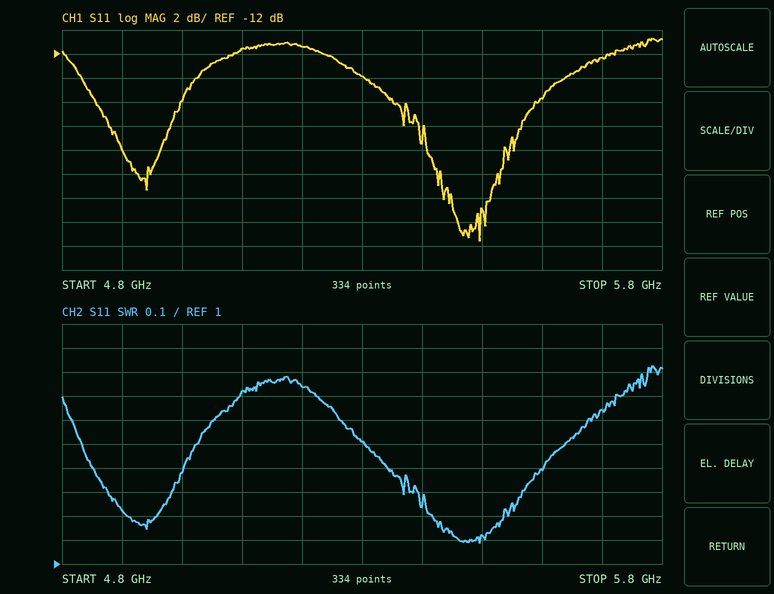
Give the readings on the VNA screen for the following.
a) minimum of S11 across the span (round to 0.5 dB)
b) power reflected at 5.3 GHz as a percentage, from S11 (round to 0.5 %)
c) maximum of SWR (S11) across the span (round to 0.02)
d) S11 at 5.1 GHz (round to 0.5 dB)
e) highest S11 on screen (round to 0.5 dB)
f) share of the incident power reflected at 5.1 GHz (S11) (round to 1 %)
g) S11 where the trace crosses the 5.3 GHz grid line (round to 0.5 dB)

-27.5 dB
4.0 %
1.82
-11.5 dB
-10.5 dB
7 %
-14.0 dB
